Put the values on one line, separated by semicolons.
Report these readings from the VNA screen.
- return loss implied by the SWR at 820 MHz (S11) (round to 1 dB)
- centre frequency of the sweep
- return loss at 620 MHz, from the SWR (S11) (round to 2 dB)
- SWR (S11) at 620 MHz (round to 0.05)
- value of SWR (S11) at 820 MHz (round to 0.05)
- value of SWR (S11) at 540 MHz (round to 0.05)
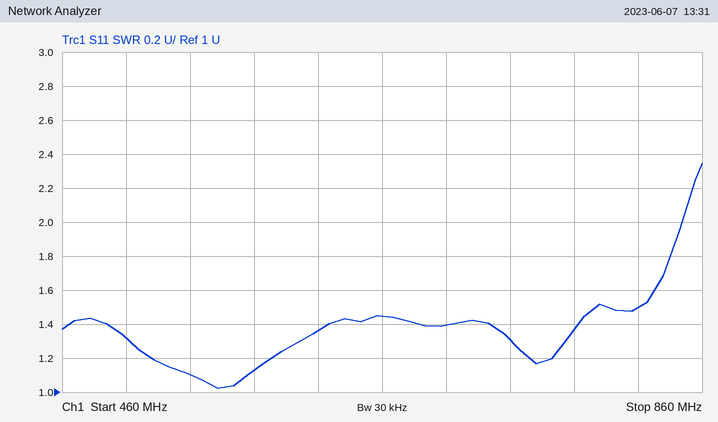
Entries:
14 dB; 660 MHz; 16 dB; 1.35; 1.50; 1.10
